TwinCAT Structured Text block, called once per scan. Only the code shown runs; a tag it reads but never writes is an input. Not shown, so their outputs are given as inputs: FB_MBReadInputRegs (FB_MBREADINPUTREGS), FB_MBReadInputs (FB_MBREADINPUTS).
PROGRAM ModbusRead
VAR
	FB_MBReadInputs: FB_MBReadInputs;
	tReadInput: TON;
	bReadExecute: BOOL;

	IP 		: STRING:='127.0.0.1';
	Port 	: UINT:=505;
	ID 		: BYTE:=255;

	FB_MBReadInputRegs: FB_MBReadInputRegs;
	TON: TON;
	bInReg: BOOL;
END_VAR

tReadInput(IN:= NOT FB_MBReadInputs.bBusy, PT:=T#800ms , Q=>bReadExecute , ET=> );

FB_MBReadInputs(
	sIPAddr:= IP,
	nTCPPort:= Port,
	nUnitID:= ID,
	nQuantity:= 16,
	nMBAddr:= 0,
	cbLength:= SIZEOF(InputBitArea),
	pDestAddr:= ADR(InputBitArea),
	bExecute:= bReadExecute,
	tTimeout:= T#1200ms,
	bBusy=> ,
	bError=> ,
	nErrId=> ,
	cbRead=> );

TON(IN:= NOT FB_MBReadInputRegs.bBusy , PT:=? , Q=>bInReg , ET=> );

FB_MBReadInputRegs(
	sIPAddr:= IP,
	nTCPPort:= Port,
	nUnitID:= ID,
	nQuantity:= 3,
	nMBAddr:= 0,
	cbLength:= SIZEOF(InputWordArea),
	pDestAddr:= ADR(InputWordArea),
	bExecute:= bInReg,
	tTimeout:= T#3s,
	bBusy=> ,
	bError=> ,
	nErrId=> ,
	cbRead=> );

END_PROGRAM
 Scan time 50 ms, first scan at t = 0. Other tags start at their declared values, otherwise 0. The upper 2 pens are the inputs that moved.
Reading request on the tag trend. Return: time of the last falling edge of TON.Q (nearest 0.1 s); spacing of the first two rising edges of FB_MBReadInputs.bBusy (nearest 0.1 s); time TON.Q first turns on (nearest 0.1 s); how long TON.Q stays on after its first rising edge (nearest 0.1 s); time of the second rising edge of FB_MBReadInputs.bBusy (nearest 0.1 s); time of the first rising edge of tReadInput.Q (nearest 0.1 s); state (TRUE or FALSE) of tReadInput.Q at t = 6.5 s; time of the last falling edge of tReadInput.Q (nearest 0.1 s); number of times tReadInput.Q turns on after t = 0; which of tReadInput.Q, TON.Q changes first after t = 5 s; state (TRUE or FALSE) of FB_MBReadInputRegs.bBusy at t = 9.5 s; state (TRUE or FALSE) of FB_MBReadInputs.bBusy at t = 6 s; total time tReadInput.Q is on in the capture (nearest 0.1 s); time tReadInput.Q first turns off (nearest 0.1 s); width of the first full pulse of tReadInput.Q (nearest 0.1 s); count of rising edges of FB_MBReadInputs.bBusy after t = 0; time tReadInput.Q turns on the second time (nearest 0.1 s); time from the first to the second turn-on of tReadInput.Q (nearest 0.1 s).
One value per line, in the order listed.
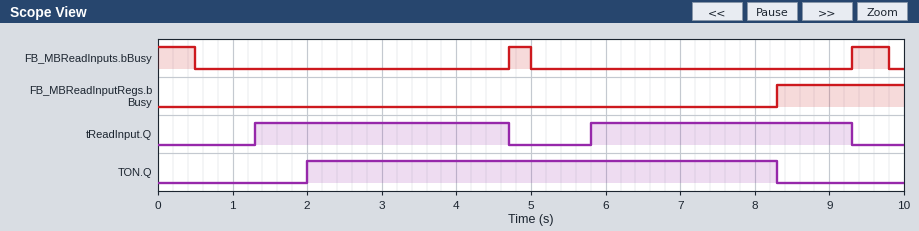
8.3 s
4.6 s
2.0 s
6.3 s
9.3 s
1.3 s
TRUE
9.3 s
2
tReadInput.Q
TRUE
FALSE
6.9 s
4.7 s
3.4 s
2
5.8 s
4.5 s
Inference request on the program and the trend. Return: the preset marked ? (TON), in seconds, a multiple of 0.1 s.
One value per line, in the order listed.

2.0 s
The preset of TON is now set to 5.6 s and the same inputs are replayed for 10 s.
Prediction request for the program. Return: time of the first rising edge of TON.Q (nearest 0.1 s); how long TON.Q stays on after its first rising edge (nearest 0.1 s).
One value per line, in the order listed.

5.6 s
2.7 s
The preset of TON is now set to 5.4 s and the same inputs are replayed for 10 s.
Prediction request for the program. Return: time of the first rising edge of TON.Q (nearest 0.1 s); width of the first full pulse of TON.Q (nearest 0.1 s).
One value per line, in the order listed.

5.4 s
2.9 s
